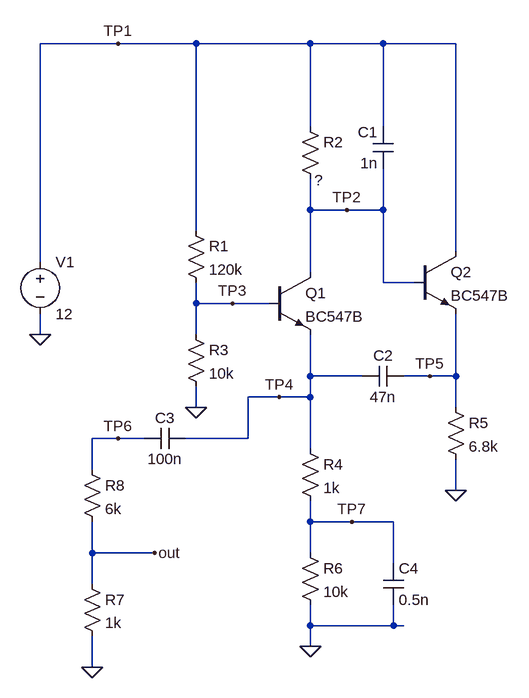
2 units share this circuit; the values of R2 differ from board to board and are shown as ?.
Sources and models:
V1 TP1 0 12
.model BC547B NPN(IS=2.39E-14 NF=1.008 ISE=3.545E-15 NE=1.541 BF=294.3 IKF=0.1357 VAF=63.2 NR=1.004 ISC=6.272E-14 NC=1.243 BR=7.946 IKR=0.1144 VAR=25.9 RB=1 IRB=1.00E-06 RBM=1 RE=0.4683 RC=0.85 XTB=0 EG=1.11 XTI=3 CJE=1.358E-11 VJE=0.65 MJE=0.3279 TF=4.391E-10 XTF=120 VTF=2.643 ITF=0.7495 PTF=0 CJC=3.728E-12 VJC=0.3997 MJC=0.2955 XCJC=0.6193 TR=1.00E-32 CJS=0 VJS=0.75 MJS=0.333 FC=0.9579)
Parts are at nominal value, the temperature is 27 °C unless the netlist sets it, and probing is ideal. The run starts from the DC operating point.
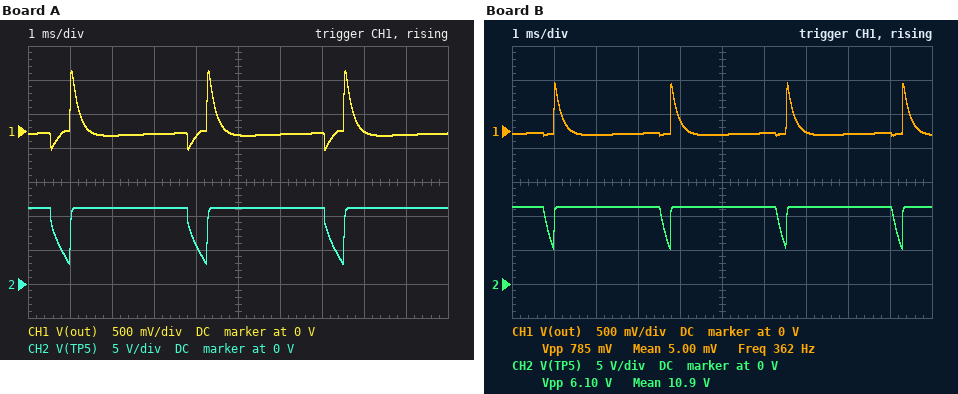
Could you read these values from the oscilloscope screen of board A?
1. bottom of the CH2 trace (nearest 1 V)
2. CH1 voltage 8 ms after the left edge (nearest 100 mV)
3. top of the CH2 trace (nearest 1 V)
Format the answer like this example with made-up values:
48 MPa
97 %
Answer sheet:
3 V
0 V
11 V
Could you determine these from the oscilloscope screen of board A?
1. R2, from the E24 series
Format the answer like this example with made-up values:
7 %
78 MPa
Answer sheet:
18 kΩ
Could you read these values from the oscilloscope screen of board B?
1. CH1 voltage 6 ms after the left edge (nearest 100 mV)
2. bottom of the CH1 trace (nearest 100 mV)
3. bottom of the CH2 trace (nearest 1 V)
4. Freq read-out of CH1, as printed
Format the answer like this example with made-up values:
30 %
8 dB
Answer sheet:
0 V
-100 mV
5 V
362 Hz
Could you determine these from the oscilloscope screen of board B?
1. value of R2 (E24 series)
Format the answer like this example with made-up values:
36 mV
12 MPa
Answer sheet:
8.2 kΩ
